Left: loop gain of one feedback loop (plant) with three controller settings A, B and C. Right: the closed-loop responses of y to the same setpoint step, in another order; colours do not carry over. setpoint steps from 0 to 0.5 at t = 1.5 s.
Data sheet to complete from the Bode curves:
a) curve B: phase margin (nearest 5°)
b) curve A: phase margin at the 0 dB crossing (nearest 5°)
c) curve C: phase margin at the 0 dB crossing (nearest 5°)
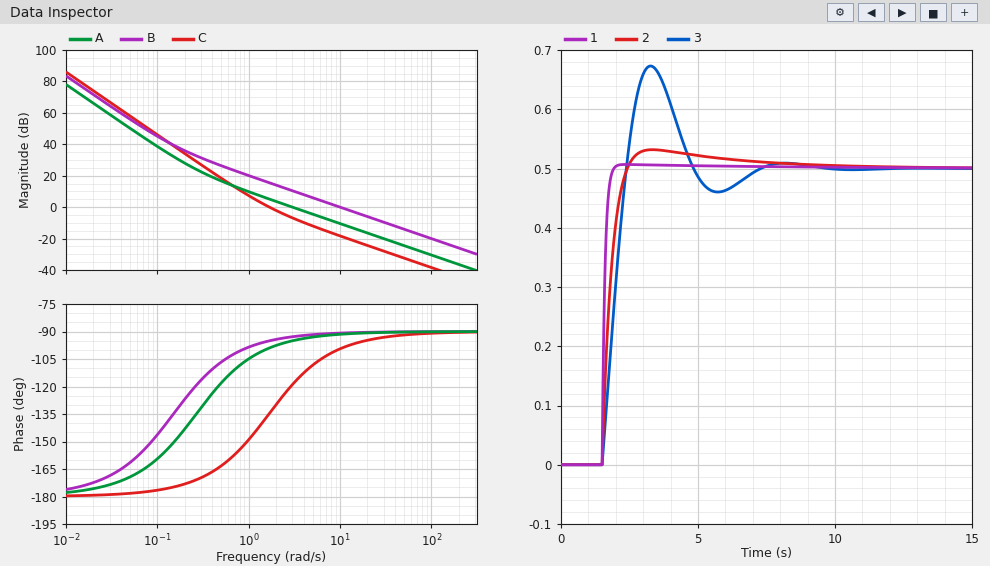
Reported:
90°
85°
45°
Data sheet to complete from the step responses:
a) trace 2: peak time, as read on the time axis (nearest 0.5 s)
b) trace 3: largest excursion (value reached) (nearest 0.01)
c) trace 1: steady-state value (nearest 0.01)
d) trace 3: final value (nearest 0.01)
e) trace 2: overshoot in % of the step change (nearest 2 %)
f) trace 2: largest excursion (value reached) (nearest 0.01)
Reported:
3.5 s
0.67
0.50
0.50
6 %
0.53
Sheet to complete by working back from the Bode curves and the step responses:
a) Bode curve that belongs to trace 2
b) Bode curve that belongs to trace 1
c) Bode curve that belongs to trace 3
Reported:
A
B
C
